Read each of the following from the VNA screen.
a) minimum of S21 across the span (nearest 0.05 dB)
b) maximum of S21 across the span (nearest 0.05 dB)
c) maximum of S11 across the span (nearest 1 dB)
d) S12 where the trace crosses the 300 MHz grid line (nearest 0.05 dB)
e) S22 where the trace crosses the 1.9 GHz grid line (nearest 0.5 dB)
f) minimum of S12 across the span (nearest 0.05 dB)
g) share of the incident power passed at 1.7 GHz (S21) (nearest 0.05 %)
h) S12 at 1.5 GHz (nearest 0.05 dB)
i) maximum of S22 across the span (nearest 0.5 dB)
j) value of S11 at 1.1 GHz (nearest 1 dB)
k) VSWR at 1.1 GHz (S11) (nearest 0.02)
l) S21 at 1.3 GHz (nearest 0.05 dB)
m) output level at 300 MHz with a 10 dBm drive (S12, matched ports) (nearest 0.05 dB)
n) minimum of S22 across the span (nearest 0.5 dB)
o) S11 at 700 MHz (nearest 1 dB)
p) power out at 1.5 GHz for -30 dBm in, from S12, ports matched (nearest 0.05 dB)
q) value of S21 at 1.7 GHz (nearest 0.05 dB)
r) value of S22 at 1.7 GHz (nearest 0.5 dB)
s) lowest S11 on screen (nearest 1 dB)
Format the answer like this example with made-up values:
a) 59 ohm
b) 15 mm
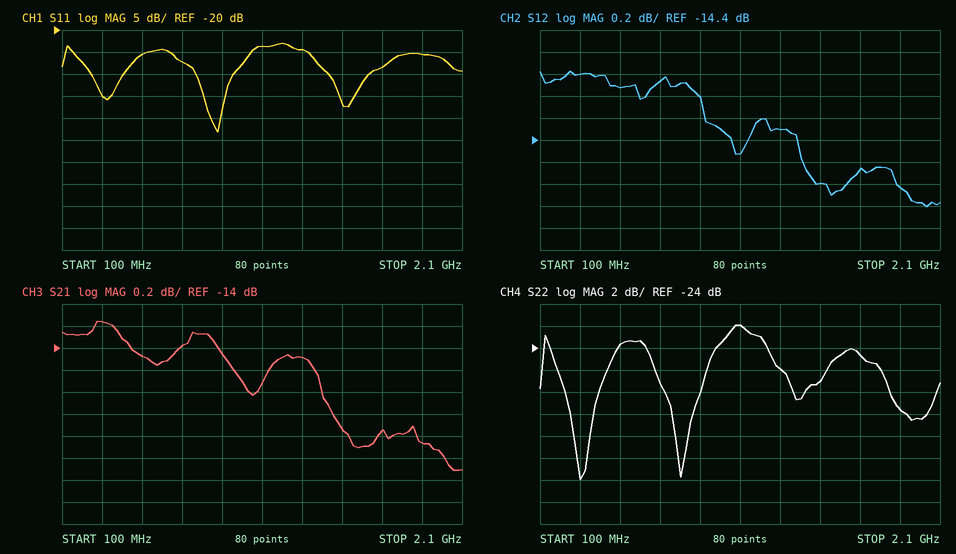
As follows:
a) -15.10 dB
b) -13.75 dB
c) -23 dB
d) -13.80 dB
e) -29.5 dB
f) -15.00 dB
g) 3.35 %
h) -14.80 dB
i) -22.0 dB
j) -24 dB
k) 1.14
l) -14.10 dB
m) -3.80 dBm
n) -36.0 dB
o) -27 dB
p) -44.80 dBm
q) -14.75 dB
r) -24.5 dB
s) -43 dB
